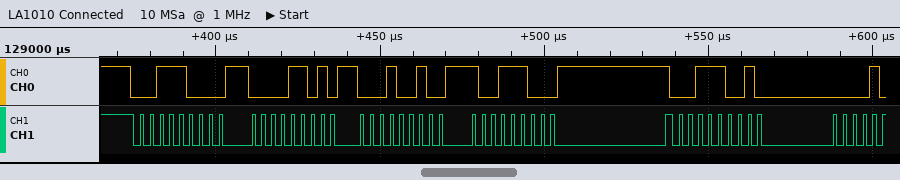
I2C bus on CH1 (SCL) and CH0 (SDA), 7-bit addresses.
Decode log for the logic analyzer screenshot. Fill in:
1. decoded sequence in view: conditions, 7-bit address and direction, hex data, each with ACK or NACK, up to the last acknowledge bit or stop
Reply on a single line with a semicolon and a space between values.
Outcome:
start, address 1C write ACK, 0D ACK, 12 ACK, 9C ACK, repeated start, address 1C read ACK
